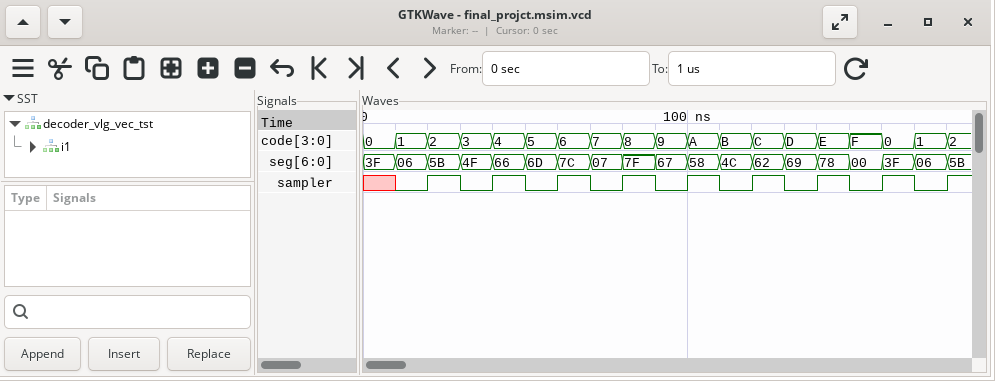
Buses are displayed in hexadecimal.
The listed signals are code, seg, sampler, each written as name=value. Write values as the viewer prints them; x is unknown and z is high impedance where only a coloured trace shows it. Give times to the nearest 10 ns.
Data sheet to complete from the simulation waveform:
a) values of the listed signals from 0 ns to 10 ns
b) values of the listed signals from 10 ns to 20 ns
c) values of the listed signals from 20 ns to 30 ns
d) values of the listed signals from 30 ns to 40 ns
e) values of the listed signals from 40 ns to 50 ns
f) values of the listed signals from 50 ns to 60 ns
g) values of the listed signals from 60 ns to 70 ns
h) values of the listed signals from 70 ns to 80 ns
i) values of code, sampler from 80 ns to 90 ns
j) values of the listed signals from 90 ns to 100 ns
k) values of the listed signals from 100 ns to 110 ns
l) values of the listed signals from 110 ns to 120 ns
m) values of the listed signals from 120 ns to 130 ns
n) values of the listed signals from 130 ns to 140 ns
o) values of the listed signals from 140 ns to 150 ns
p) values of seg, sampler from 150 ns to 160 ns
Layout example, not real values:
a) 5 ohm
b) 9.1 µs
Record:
a) code=0, seg=3F, sampler=x
b) code=1, seg=06, sampler=0
c) code=2, seg=5B, sampler=1
d) code=3, seg=4F, sampler=0
e) code=4, seg=66, sampler=1
f) code=5, seg=6D, sampler=0
g) code=6, seg=7C, sampler=1
h) code=7, seg=07, sampler=0
i) code=8, sampler=1
j) code=9, seg=67, sampler=0
k) code=A, seg=58, sampler=1
l) code=B, seg=4C, sampler=0
m) code=C, seg=62, sampler=1
n) code=D, seg=69, sampler=0
o) code=E, seg=78, sampler=1
p) seg=00, sampler=0
